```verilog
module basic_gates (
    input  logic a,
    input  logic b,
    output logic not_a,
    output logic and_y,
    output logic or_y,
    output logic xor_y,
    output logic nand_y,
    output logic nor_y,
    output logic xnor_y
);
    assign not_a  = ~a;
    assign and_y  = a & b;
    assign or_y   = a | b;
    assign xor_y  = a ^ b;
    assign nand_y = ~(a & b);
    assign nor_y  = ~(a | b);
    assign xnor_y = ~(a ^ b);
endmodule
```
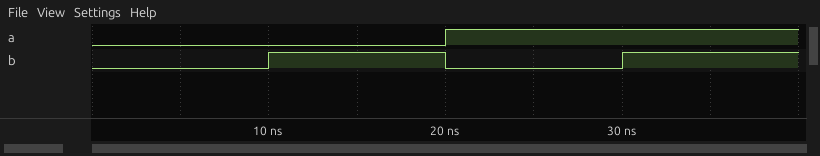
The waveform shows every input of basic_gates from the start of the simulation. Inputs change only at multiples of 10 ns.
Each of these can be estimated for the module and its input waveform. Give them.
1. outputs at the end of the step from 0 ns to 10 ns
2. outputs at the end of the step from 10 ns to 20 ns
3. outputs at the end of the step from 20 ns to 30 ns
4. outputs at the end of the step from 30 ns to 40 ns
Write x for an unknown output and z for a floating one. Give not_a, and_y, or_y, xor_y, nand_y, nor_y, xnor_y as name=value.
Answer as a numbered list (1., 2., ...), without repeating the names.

1. not_a=1, and_y=0, or_y=0, xor_y=0, nand_y=1, nor_y=1, xnor_y=1
2. not_a=1, and_y=0, or_y=1, xor_y=1, nand_y=1, nor_y=0, xnor_y=0
3. not_a=0, and_y=0, or_y=1, xor_y=1, nand_y=1, nor_y=0, xnor_y=0
4. not_a=0, and_y=1, or_y=1, xor_y=0, nand_y=0, nor_y=0, xnor_y=1
